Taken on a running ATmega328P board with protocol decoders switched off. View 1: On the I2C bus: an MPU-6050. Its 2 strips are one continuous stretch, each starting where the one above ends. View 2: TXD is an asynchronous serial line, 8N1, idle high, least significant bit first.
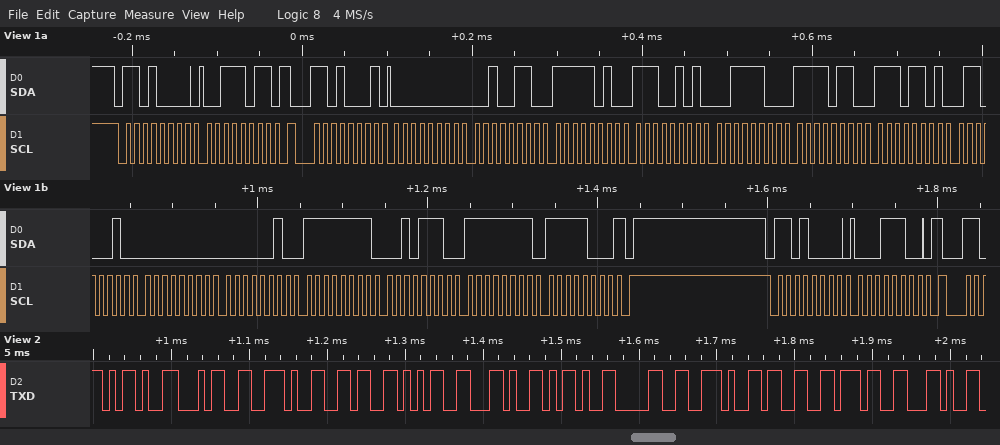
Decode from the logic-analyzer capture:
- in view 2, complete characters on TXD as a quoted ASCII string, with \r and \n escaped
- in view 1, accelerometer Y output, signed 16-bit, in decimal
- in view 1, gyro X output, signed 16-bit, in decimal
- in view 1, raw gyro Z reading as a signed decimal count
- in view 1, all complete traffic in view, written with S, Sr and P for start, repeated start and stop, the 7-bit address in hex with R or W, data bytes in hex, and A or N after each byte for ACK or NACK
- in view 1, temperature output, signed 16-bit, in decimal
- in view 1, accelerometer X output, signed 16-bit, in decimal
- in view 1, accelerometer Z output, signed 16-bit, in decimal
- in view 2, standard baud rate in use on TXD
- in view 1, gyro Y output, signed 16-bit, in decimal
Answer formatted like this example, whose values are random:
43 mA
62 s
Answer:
"-4.65,-0.37,"
-1307
2
-8
S 68W A 3B A Sr 68R A 00 A 26 A FA A E5 A 3C A F6 A ED A 62 A 00 A 02 A FF A 2E A FF A F8 N P S 68W A 1C A
-4766
38
15606
115200 baud
-210
